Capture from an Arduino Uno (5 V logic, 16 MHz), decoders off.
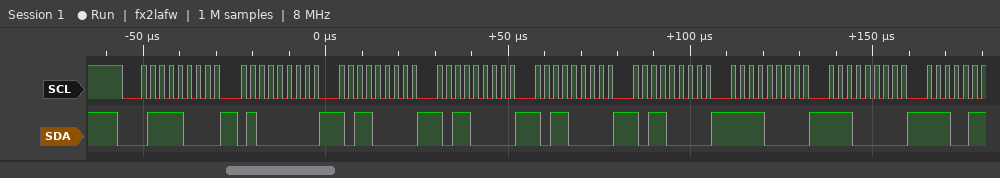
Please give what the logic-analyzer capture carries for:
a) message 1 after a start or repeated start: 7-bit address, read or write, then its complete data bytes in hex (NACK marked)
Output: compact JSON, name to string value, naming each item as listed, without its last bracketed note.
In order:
{"message 1 after a start or repeated start: 7-bit address, read or write, then its complete data bytes in hex": "0x3C write: 40 B0 B0 B0 B0 F0 E0"}
